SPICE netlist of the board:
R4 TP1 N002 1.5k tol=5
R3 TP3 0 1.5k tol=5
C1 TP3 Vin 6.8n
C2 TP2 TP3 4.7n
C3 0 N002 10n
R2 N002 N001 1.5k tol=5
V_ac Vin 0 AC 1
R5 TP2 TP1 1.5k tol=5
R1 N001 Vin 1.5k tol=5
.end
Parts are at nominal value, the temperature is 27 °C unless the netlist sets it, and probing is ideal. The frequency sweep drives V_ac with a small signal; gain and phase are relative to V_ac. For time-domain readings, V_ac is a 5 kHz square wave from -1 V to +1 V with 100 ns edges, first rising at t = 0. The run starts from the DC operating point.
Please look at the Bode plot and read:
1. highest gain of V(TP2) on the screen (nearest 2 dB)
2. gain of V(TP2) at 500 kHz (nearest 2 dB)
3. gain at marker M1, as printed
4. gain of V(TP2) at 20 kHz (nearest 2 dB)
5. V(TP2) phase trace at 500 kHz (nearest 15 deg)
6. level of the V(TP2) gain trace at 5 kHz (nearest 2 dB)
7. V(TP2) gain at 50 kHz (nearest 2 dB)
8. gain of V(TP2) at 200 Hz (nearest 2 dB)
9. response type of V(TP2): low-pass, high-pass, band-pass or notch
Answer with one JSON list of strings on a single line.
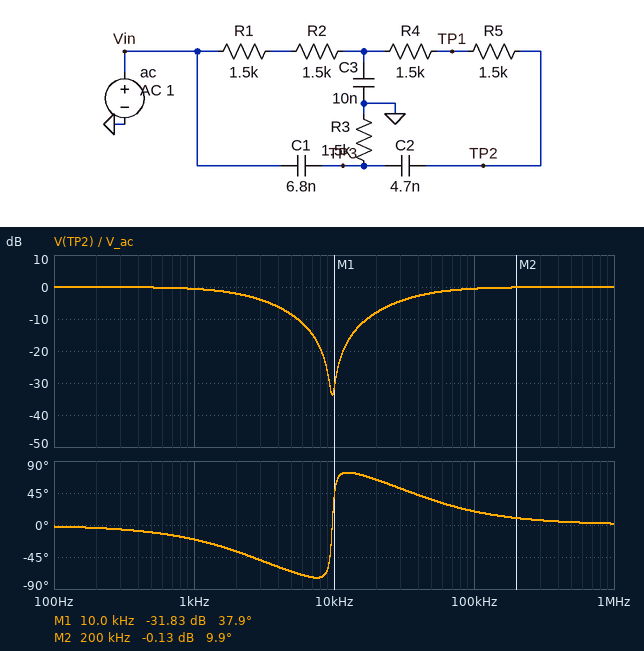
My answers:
["0 dB", "0 dB", "-31.83 dB", "-8 dB", "0 deg", "-8 dB", "-2 dB", "0 dB", "notch"]
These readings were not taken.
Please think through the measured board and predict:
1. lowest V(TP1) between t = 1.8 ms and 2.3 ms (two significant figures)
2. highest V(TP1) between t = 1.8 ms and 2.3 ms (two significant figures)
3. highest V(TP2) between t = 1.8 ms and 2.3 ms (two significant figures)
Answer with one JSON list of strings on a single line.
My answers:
["-730 mV", "730 mV", "1.3 V"]
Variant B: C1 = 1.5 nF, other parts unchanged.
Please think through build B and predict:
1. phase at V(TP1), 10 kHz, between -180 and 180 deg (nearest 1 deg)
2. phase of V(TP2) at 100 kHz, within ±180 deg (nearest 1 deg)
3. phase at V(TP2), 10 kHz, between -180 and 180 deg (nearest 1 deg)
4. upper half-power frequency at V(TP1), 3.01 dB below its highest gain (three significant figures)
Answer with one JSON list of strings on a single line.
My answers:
["-66 deg", "51 deg", "-92 deg", "2.95 kHz"]
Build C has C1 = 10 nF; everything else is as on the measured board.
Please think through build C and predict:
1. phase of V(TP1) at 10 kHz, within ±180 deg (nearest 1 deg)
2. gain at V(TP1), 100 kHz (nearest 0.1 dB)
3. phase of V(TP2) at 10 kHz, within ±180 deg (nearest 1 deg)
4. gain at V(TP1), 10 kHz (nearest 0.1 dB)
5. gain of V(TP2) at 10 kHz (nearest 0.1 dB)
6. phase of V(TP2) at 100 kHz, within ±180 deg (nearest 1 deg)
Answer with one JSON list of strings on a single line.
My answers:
["-22 deg", "-6.4 dB", "51 deg", "-13.8 dB", "-18.8 dB", "15 deg"]
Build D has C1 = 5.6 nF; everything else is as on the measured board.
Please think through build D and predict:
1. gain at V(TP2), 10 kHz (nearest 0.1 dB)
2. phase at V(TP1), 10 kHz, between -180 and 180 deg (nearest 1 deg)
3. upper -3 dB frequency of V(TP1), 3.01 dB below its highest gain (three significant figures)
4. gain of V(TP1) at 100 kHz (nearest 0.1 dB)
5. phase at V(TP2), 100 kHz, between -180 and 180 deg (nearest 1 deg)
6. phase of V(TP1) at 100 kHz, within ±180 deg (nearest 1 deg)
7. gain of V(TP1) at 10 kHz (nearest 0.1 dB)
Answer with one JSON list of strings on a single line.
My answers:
["-33.3 dB", "-46 deg", "2.75 kHz", "-6.7 dB", "22 deg", "16 deg", "-14.3 dB"]
